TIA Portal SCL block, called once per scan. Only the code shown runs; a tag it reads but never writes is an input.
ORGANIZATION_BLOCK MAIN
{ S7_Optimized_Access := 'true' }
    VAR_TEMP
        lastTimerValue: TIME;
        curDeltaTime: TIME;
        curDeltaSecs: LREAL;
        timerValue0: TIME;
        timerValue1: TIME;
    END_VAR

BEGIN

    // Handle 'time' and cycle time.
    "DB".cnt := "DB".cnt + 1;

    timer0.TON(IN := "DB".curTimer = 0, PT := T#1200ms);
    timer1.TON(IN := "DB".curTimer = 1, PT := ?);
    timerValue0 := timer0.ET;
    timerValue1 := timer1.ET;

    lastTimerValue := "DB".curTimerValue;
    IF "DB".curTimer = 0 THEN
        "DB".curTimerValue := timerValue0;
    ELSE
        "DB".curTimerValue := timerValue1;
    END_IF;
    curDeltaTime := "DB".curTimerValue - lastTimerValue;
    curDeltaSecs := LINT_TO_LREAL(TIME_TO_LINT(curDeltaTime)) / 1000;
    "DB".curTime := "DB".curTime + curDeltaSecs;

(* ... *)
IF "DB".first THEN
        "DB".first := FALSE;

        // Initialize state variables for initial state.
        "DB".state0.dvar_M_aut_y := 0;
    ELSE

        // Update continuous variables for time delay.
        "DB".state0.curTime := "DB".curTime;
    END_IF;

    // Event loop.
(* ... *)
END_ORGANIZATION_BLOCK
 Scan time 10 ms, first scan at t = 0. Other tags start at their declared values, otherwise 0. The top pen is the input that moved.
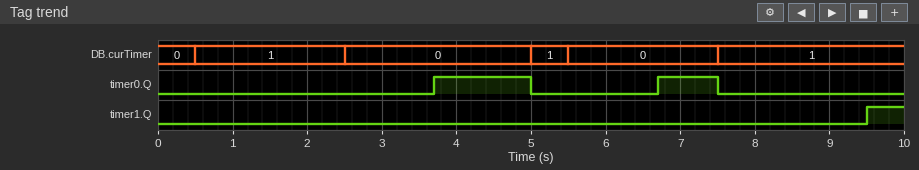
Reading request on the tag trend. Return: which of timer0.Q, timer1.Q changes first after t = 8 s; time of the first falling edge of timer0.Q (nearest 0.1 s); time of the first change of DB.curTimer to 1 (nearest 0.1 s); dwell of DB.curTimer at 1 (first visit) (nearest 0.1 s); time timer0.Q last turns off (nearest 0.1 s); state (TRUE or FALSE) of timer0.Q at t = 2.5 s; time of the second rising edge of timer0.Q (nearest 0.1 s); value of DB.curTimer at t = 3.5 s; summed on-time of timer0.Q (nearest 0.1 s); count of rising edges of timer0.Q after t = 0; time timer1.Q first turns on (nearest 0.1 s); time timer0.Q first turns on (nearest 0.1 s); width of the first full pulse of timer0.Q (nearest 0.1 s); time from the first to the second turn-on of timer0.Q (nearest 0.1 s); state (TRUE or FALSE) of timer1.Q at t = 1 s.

timer1.Q
5.0 s
0.5 s
2.0 s
7.5 s
FALSE
6.7 s
0
2.1 s
2
9.5 s
3.7 s
1.3 s
3.0 s
FALSE
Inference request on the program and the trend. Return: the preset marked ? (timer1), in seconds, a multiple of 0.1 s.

2.0 s
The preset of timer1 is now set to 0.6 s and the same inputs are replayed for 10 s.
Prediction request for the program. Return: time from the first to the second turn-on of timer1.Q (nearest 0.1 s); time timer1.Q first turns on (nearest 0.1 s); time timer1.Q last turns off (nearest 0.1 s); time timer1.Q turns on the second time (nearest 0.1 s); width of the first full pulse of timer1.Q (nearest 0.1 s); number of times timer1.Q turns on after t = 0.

7.0 s
1.1 s
2.5 s
8.1 s
1.4 s
2
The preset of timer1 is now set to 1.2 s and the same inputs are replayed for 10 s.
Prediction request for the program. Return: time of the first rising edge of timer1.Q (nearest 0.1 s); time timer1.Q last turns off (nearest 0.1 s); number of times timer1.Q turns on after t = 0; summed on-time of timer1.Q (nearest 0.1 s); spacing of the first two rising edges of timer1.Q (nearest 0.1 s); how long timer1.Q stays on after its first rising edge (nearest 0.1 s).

1.7 s
2.5 s
2
2.1 s
7.0 s
0.8 s
